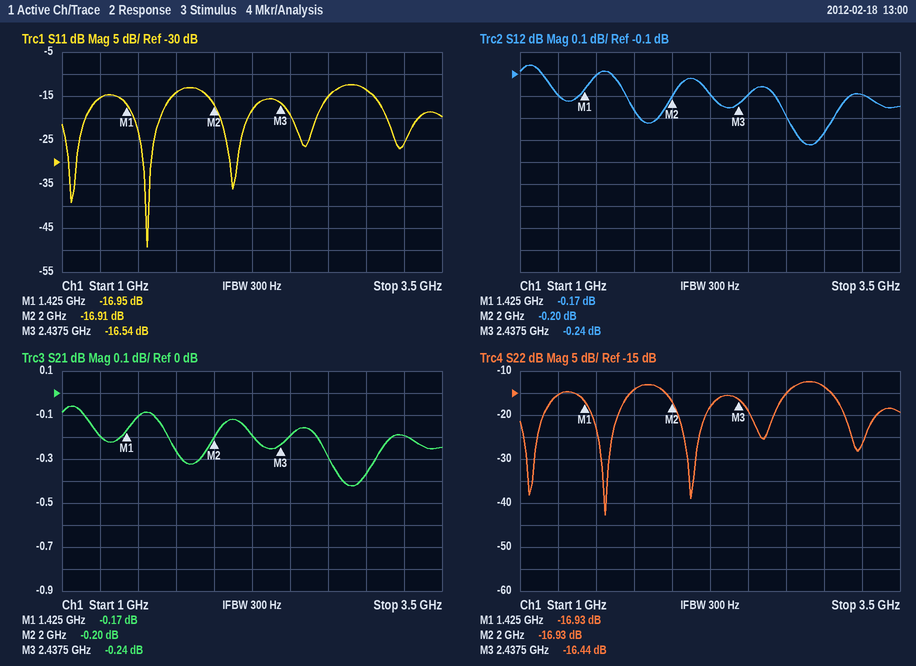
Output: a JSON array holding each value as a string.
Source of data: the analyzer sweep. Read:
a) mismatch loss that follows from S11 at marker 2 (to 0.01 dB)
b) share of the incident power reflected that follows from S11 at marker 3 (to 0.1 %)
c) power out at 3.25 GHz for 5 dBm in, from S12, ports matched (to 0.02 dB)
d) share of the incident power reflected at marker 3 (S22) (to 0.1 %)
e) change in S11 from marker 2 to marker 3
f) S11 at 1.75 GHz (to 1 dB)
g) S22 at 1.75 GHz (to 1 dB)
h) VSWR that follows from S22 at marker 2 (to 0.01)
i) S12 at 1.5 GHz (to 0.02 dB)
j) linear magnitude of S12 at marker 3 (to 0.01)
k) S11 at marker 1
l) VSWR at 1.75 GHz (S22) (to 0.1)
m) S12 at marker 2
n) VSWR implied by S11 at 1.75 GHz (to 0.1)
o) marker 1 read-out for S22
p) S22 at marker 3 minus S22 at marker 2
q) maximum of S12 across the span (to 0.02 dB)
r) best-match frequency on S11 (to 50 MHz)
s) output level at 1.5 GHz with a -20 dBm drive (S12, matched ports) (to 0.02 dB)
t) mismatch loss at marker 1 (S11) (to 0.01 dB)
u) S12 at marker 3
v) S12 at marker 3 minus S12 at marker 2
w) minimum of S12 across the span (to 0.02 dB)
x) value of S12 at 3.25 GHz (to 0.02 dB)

["0.09 dB", "2.2 %", "4.80 dBm", "2.3 %", "0.37 dB", "-14 dB", "-14 dB", "1.33", "-0.10 dB", "0.97", "-16.95 dB", "1.5", "-0.20 dB", "1.5", "-16.93 dB", "0.49 dB", "-0.06 dB", "1.55 GHz", "-20.10 dBm", "0.09 dB", "-0.24 dB", "-0.04 dB", "-0.42 dB", "-0.20 dB"]
